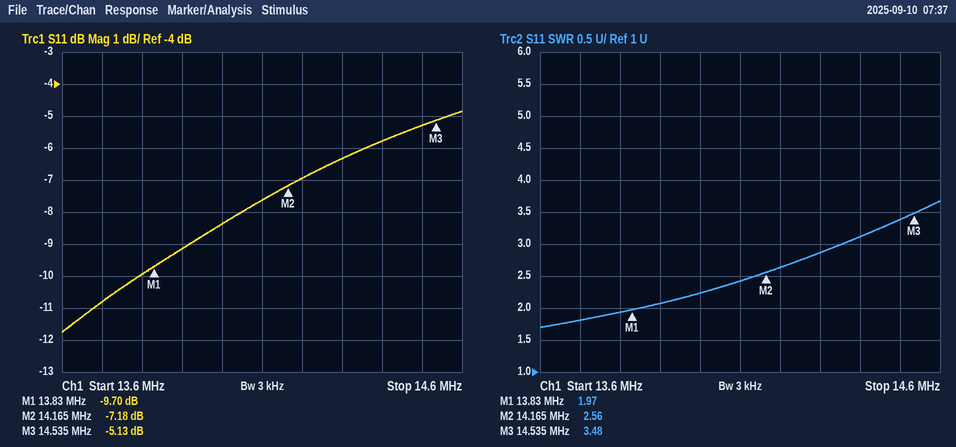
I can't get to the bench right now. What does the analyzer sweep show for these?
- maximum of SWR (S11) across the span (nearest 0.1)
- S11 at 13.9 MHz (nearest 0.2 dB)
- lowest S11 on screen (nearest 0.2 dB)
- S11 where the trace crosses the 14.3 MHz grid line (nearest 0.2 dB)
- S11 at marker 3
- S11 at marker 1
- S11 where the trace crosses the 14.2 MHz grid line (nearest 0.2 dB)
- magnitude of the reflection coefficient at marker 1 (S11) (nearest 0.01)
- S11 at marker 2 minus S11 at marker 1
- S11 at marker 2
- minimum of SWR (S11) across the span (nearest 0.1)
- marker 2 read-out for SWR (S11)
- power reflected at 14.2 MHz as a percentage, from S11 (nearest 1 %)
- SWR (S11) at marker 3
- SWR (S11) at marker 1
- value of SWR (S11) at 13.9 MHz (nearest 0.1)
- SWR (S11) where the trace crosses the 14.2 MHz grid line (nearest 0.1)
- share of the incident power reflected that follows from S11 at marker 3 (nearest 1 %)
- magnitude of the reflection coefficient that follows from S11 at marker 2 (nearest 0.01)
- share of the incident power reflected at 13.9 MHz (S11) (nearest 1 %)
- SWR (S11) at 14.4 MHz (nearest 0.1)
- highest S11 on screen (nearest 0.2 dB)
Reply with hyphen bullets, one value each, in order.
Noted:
- 3.7
- -9.2 dB
- -11.8 dB
- -6.4 dB
- -5.13 dB
- -9.70 dB
- -7.0 dB
- 0.33
- 2.52 dB
- -7.18 dB
- 1.7
- 2.56
- 20 %
- 3.48
- 1.97
- 2.1
- 2.6
- 31 %
- 0.44
- 12 %
- 3.1
- -4.8 dB
